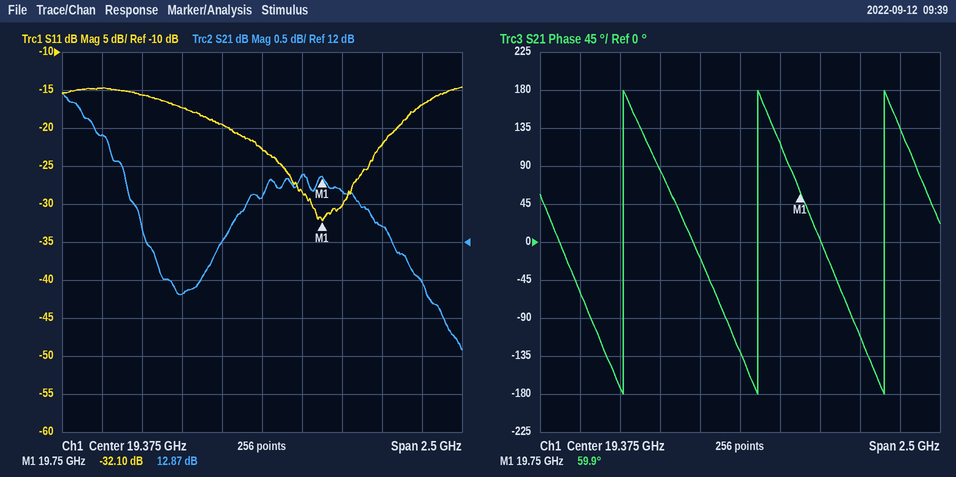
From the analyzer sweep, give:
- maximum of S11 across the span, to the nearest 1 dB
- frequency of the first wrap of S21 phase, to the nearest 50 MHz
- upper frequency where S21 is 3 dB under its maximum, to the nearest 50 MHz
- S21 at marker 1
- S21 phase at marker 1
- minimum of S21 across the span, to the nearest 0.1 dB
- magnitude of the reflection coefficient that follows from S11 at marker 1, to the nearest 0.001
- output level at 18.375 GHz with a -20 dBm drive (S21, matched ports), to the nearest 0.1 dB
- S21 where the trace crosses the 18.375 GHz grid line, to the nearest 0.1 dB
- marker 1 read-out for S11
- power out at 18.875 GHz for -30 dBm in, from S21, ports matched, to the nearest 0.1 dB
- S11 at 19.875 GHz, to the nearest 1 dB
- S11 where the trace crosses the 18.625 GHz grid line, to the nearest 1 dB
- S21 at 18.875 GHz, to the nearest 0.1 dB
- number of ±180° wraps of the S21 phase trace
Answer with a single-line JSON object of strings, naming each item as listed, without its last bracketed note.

{"maximum of S11 across the span, to the nearest 1 dB": "-15 dB", "frequency of the first wrap of S21 phase, to the nearest 50 MHz": "18.65 GHz", "upper frequency where S21 is 3 dB under its maximum, to the nearest 50 MHz": "20.50 GHz", "S21 at marker 1": "12.87 dB", "S21 phase at marker 1": "59.9°", "minimum of S21 across the span, to the nearest 0.1 dB": "10.6 dB", "magnitude of the reflection coefficient that follows from S11 at marker 1, to the nearest 0.001": "0.025", "output level at 18.375 GHz with a -20 dBm drive (S21, matched ports), to the nearest 0.1 dB": "-6.6 dBm", "S21 where the trace crosses the 18.375 GHz grid line, to the nearest 0.1 dB": "13.4 dB", "marker 1 read-out for S11": "-32.10 dB", "power out at 18.875 GHz for -30 dBm in, from S21, ports matched, to the nearest 0.1 dB": "-18.7 dBm", "S11 at 19.875 GHz, to the nearest 1 dB": "-30 dB", "S11 where the trace crosses the 18.625 GHz grid line, to the nearest 1 dB": "-16 dB", "S21 at 18.875 GHz, to the nearest 0.1 dB": "11.3 dB", "number of ±180° wraps of the S21 phase trace": "3"}
